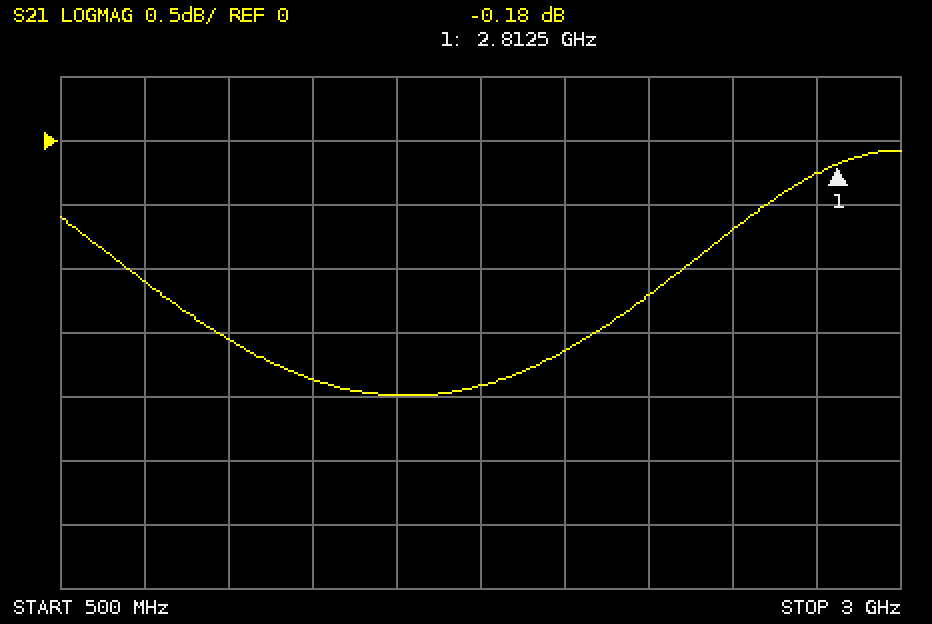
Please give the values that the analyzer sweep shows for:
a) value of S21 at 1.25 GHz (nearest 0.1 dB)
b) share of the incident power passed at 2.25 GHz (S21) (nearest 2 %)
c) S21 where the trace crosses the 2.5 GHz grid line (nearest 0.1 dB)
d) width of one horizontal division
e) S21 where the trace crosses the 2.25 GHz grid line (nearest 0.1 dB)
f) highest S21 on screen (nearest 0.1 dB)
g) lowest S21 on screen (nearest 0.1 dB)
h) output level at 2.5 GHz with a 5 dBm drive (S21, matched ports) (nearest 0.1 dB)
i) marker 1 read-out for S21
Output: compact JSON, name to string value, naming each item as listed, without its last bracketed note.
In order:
{"value of S21 at 1.25 GHz": "-1.9 dB", "share of the incident power passed at 2.25 GHz (S21)": "76 %", "S21 where the trace crosses the 2.5 GHz grid line": "-0.7 dB", "width of one horizontal division": "250 MHz", "S21 where the trace crosses the 2.25 GHz grid line": "-1.2 dB", "highest S21 on screen": "-0.1 dB", "lowest S21 on screen": "-2.0 dB", "output level at 2.5 GHz with a 5 dBm drive (S21, matched ports)": "4.3 dBm", "marker 1 read-out for S21": "-0.18 dB"}
